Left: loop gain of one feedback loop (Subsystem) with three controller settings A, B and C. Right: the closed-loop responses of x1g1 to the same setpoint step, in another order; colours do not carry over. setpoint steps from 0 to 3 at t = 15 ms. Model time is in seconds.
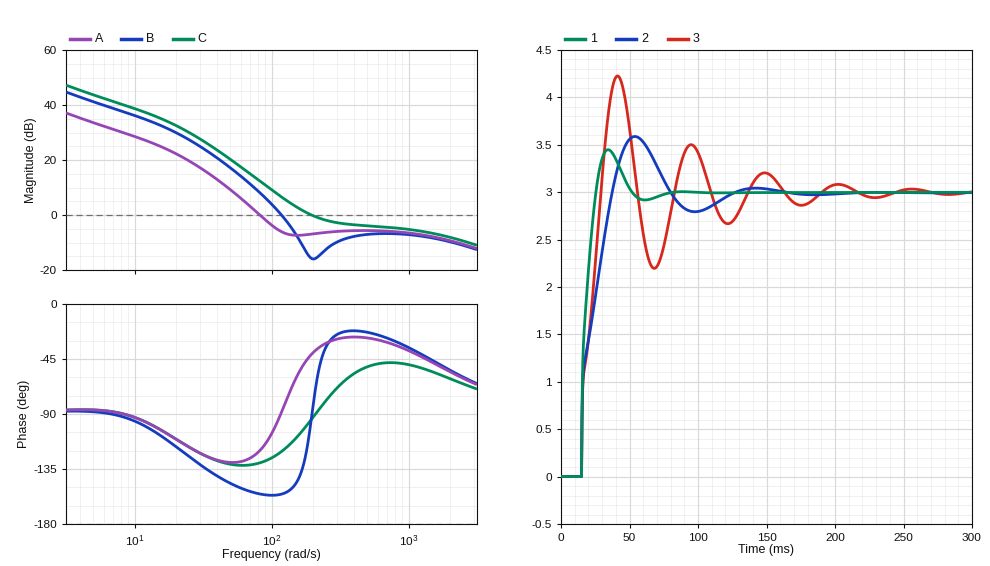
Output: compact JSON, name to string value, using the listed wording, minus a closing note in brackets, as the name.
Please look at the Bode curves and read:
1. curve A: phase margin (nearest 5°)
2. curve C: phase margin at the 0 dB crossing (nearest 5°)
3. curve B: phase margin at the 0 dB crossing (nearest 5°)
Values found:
{"curve A: phase margin": "60°", "curve C: phase margin at the 0 dB crossing": "85°", "curve B: phase margin at the 0 dB crossing": "25°"}
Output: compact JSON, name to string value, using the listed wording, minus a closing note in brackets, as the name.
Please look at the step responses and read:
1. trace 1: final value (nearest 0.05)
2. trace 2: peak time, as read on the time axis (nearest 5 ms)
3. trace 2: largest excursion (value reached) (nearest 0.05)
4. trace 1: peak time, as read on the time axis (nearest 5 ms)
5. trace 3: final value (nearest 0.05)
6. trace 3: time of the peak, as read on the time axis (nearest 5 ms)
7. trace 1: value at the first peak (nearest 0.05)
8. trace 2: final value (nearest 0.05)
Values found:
{"trace 1: final value": "3.00", "trace 2: peak time, as read on the time axis": "55 ms", "trace 2: largest excursion (value reached)": "3.60", "trace 1: peak time, as read on the time axis": "35 ms", "trace 3: final value": "3.00", "trace 3: time of the peak, as read on the time axis": "40 ms", "trace 1: value at the first peak": "3.45", "trace 2: final value": "3.00"}
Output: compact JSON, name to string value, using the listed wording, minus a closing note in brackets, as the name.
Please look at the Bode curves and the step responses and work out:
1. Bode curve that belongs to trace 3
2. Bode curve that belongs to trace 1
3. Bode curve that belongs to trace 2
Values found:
{"Bode curve that belongs to trace 3": "B", "Bode curve that belongs to trace 1": "C", "Bode curve that belongs to trace 2": "A"}
